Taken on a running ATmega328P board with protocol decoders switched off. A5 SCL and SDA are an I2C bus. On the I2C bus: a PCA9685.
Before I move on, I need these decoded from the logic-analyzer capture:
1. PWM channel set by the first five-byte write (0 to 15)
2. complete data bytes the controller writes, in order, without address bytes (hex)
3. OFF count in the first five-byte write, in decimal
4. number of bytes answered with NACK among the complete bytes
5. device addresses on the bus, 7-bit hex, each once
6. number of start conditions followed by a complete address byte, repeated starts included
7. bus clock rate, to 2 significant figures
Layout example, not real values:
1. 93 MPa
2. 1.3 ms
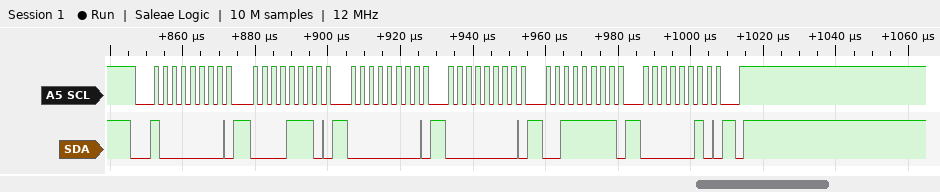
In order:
1. 2
2. 0E 00 00 3F 02
3. 575
4. 0
5. 0x40
6. 1
7. 400 kHz
